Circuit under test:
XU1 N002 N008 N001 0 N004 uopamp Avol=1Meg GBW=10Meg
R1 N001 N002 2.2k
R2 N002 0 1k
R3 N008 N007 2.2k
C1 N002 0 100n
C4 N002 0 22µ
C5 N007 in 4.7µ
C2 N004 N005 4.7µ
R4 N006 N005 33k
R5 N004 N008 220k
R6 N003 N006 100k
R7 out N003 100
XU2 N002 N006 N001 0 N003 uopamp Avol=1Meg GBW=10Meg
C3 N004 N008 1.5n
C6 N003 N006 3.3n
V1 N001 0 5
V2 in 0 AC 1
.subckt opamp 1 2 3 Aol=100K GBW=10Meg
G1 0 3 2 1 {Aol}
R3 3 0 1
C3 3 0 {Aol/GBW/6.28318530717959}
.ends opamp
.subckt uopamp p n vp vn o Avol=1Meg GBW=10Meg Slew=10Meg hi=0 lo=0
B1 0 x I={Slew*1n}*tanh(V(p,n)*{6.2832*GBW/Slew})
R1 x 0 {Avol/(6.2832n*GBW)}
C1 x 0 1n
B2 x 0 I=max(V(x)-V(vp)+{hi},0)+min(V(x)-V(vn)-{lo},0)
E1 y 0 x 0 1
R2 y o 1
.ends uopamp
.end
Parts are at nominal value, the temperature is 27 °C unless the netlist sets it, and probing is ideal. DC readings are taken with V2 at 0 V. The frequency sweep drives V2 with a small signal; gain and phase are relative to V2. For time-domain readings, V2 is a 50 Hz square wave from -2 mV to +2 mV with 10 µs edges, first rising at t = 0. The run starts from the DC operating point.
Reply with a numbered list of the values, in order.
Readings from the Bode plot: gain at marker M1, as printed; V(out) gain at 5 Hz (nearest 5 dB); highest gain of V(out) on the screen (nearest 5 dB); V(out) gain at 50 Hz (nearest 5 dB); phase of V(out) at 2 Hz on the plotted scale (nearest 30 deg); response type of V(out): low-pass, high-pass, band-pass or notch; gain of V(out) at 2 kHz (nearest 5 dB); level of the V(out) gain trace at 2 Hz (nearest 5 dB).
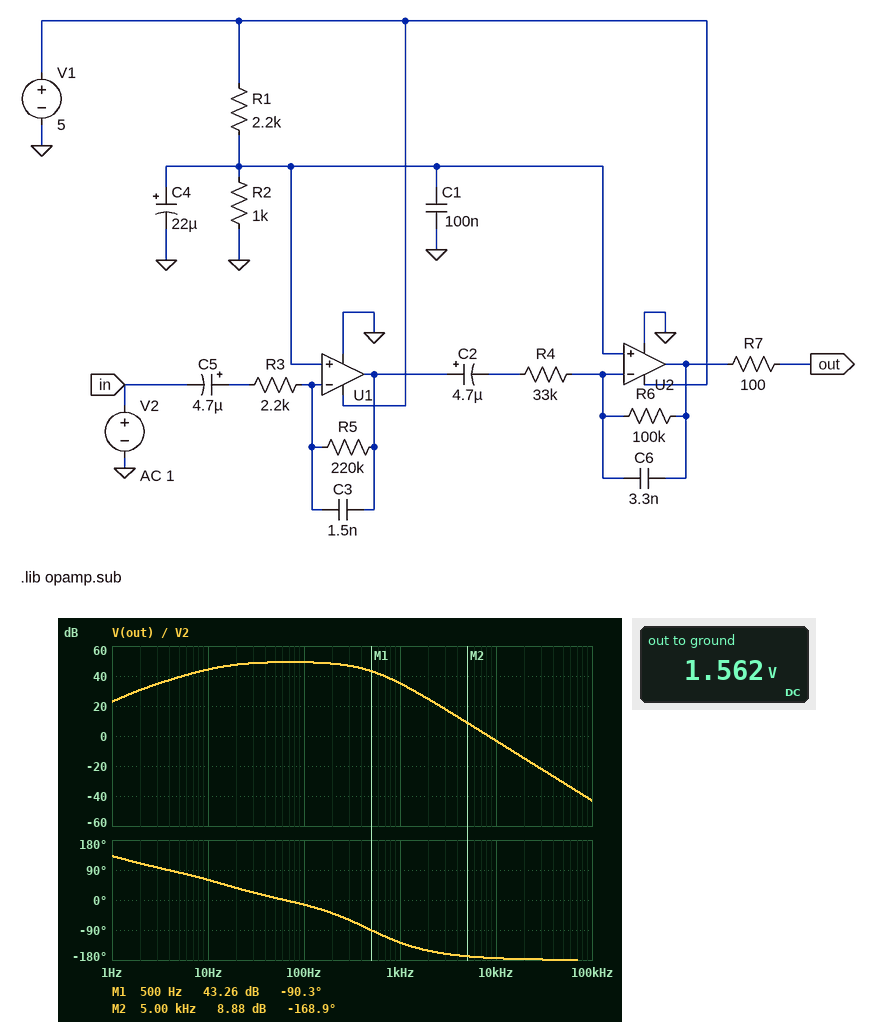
1. 43.26 dB
2. 40 dB
3. 50 dB
4. 50 dB
5. 120 deg
6. band-pass
7. 25 dB
8. 30 dB
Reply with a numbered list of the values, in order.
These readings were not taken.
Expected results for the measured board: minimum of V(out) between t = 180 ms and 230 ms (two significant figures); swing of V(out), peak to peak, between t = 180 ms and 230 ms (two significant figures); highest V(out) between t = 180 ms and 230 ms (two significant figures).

1. 790 mV
2. 1.5 V
3. 2.3 V
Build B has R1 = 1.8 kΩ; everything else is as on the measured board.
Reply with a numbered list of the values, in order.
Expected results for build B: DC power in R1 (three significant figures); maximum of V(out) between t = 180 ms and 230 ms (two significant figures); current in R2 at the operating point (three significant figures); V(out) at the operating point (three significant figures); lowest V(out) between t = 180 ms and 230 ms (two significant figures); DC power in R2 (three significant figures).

1. 5.74 mW
2. 2.5 V
3. 1.79 mA
4. 1.79 V
5. 1.0 V
6. 3.19 mW
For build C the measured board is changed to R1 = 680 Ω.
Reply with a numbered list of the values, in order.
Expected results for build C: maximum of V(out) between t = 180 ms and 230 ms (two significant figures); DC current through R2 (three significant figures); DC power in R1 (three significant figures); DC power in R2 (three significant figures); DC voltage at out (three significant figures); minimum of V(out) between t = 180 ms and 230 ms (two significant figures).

1. 3.7 V
2. 2.98 mA
3. 6.02 mW
4. 8.86 mW
5. 2.98 V
6. 2.2 V
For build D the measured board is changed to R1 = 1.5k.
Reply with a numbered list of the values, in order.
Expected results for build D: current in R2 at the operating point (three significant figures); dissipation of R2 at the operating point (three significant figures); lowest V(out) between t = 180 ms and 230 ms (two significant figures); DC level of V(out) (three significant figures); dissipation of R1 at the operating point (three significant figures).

1. 2.00 mA
2. 4.00 mW
3. 1.2 V
4. 2.00 V
5. 6.00 mW
